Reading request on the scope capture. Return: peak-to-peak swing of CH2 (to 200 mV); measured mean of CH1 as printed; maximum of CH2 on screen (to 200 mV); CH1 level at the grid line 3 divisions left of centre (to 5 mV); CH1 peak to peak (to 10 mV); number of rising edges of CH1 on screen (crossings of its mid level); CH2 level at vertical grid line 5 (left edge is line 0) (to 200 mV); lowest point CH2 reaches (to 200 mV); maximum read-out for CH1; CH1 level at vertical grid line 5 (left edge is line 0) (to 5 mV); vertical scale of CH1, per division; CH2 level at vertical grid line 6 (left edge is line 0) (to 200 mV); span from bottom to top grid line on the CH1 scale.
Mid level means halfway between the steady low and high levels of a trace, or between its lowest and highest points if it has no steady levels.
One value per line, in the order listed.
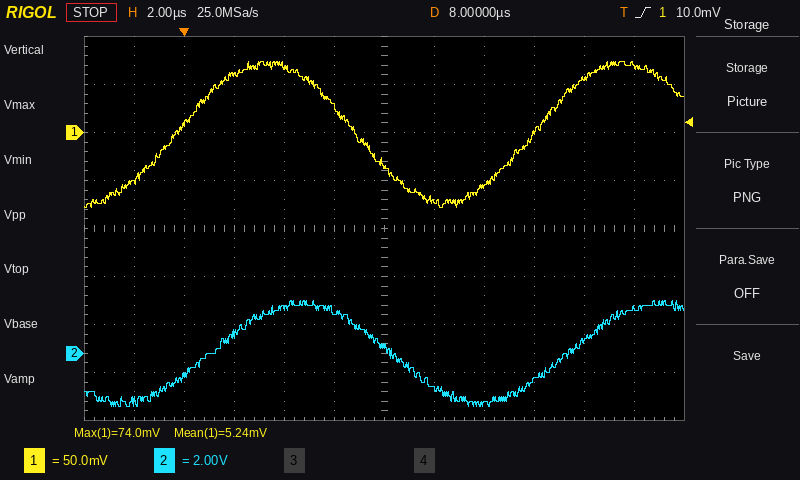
4.4 V
5.24 mV
2.2 V
60 mV
150 mV
2
1.8 V
-2.2 V
74.0 mV
25 mV
50 mV
200 mV
400 mV
